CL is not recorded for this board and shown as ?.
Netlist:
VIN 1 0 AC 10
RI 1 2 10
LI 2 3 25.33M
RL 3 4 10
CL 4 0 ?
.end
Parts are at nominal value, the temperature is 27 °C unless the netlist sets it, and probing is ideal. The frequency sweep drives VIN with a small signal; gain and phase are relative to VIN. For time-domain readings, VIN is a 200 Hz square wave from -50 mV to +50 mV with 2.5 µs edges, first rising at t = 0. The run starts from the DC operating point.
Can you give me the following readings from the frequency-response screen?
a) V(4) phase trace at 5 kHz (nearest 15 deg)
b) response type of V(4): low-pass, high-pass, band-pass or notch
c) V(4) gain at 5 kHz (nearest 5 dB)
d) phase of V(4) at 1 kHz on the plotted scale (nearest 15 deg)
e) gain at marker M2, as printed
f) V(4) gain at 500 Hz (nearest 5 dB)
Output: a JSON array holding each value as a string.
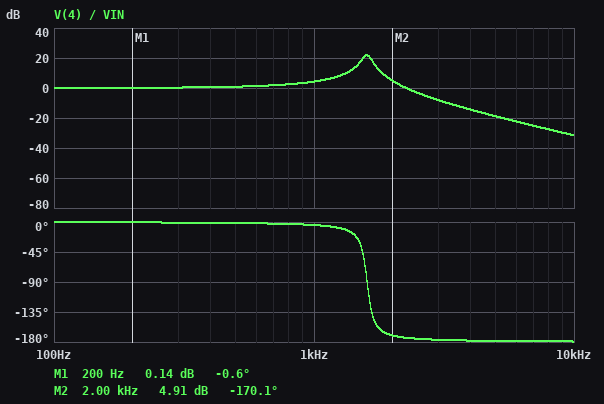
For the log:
["-180 deg", "low-pass", "-20 dB", "0 deg", "4.91 dB", "0 dB"]
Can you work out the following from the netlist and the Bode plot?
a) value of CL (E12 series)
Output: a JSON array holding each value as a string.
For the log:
["390 nF"]
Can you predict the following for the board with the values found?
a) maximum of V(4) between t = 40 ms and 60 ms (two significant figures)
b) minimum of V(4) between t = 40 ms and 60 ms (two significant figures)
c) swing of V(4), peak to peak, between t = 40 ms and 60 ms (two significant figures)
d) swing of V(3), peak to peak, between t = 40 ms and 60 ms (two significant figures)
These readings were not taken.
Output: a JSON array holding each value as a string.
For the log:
["110 mV", "-110 mV", "230 mV", "230 mV"]
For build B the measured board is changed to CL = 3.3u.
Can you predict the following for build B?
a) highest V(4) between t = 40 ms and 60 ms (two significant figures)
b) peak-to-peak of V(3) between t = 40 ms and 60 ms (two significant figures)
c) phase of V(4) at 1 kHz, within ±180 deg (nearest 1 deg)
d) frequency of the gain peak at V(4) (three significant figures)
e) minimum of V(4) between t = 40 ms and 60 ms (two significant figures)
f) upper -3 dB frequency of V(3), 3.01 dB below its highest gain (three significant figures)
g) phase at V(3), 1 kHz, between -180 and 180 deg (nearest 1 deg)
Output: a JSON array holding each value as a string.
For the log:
["130 mV", "270 mV", "-170 deg", "543 Hz", "-130 mV", "603 Hz", "-158 deg"]
